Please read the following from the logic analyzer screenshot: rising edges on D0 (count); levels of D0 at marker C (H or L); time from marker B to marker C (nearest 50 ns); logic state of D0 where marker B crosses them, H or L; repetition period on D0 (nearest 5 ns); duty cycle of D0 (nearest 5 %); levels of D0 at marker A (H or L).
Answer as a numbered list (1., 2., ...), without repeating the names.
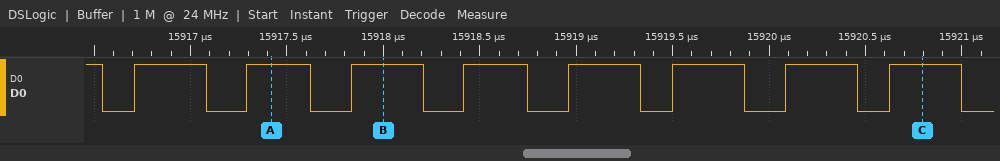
1. 8
2. D0=H
3. 2800 ns
4. D0=H
5. 560 ns
6. 65 %
7. D0=H
